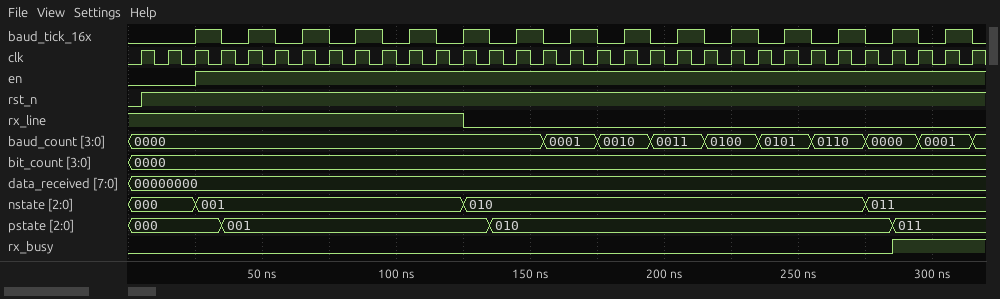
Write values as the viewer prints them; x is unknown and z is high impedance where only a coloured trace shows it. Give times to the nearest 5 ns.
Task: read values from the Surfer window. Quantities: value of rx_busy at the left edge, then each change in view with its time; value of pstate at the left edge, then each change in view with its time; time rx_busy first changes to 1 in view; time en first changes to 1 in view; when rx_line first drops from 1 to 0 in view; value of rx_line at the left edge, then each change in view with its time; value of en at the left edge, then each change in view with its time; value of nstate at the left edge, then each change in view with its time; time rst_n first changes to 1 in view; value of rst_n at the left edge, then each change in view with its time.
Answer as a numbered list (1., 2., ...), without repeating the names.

1. 0, 1 at 285 ns
2. 000, 001 at 35 ns, 010 at 135 ns, 011 at 285 ns
3. 285 ns
4. 25 ns
5. 125 ns
6. 1, 0 at 125 ns
7. 0, 1 at 25 ns
8. 000, 001 at 25 ns, 010 at 125 ns, 011 at 275 ns
9. 5 ns
10. 0, 1 at 5 ns
